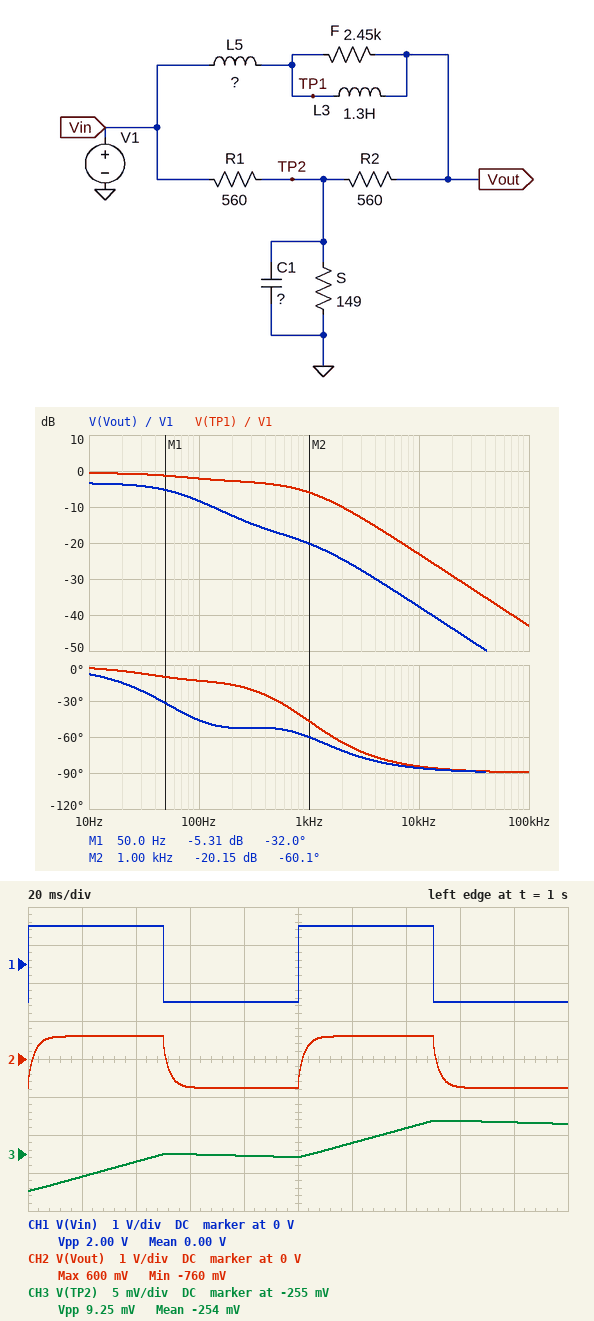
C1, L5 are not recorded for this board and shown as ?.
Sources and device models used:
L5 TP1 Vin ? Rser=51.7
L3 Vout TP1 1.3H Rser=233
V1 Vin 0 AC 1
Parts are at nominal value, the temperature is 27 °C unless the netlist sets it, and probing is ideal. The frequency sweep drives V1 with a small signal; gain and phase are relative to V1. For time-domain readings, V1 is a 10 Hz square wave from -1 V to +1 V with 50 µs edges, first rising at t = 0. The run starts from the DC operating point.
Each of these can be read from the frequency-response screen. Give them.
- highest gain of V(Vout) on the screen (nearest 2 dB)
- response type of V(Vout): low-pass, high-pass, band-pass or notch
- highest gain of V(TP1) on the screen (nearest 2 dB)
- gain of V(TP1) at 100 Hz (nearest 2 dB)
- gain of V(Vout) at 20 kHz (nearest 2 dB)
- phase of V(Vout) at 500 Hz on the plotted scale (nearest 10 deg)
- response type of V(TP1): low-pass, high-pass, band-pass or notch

-4 dB
low-pass
0 dB
-2 dB
-44 dB
-50 deg
low-pass
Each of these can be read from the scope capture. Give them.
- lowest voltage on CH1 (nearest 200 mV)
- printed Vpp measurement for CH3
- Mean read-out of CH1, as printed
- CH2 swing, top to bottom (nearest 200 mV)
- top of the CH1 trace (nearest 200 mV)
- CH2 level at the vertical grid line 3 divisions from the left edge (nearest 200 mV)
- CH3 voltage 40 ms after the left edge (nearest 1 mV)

-1.0 V
9.25 mV
0.00 V
1.4 V
1.0 V
-800 mV
-256 mV
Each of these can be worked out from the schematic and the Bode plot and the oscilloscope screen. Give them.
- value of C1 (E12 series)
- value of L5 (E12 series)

56 mF
680 mH
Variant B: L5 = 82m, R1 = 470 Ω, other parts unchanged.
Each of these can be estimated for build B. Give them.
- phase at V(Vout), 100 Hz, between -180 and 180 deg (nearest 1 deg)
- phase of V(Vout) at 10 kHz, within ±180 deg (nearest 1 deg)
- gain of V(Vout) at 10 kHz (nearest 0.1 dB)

-34 deg
-60 deg
-20.7 dB
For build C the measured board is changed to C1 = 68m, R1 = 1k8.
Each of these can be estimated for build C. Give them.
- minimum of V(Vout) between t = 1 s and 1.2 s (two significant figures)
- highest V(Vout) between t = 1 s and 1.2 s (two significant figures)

-740 mV
620 mV
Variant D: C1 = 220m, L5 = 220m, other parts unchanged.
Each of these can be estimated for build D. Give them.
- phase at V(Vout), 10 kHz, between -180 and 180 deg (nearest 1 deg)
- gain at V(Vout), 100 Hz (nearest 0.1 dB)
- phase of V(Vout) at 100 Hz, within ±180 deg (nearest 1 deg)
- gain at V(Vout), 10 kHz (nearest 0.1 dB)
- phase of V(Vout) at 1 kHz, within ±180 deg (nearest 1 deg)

-78 deg
-7.1 dB
-37 deg
-28.1 dB
-36 deg
